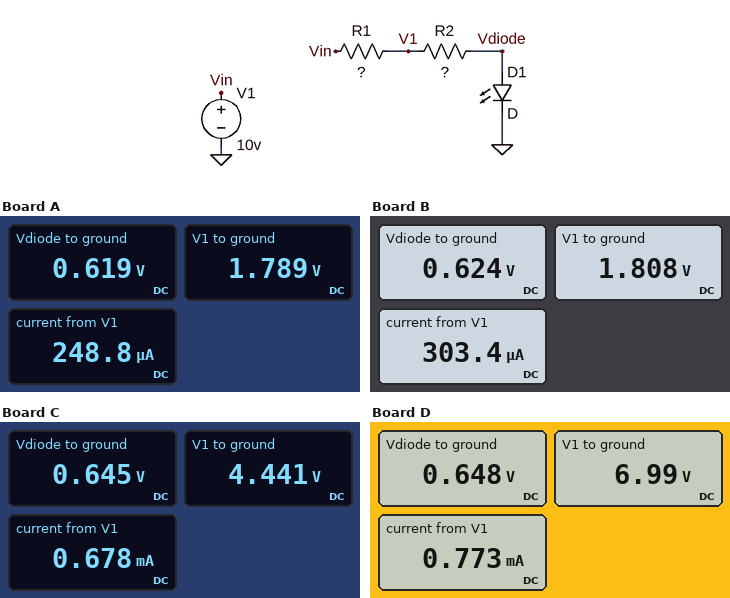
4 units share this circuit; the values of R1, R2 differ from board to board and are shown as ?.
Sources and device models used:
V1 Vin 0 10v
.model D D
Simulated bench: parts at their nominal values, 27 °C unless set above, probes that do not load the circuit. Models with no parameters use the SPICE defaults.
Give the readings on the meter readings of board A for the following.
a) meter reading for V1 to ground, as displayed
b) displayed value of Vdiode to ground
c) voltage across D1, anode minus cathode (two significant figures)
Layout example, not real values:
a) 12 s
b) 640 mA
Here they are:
a) 1.789 V
b) 0.619 V
c) 620 mV
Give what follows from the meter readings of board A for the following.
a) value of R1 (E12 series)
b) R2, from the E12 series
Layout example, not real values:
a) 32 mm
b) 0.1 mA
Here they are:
a) 33 kΩ
b) 4.7 kΩ
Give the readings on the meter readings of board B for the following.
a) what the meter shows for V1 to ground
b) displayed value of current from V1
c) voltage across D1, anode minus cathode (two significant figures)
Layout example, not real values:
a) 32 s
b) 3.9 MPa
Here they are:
a) 1.808 V
b) 303.4 µA
c) 620 mV
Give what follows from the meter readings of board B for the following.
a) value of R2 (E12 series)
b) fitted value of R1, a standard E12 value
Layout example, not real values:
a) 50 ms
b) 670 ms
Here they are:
a) 3.9 kΩ
b) 27 kΩ
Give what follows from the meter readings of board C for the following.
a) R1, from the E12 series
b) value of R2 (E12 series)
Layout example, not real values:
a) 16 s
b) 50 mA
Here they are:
a) 8.2 kΩ
b) 5.6 kΩ
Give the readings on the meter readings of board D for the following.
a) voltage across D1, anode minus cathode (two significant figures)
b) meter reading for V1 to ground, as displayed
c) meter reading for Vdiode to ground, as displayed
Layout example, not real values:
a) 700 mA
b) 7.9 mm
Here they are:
a) 650 mV
b) 6.99 V
c) 0.648 V
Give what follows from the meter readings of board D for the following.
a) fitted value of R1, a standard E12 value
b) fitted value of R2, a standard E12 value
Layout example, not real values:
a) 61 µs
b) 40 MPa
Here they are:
a) 3.9 kΩ
b) 8.2 kΩ
